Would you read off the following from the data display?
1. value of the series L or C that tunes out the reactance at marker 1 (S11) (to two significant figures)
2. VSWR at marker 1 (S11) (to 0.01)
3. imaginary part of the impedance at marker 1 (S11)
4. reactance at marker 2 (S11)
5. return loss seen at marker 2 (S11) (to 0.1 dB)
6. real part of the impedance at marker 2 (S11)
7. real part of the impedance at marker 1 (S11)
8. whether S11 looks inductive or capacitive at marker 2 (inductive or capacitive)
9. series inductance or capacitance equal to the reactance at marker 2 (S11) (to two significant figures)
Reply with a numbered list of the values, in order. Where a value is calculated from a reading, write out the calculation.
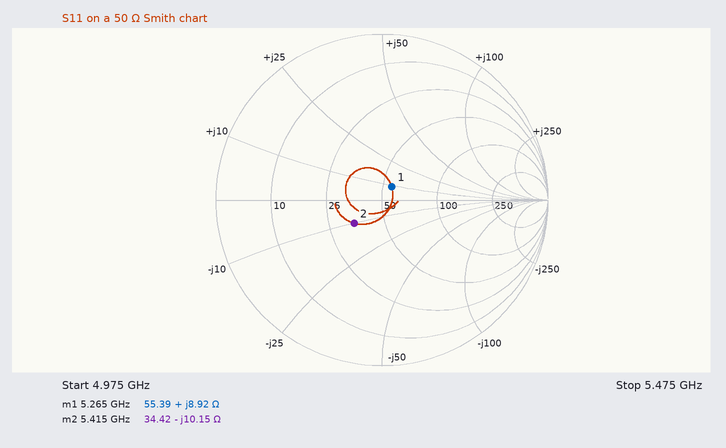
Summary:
1. C = 1/(2π × 5.265 GHz × 8.92 Ω) ≈ 3.4 pF
2. 1.22
3. +8.92 Ω
4. -10.15 Ω
5. 13.2 dB
6. 34.42 Ω
7. 55.39 Ω
8. capacitive
9. C = 1/(2π × 5.415 GHz × 10.15 Ω) ≈ 2.9 pF
